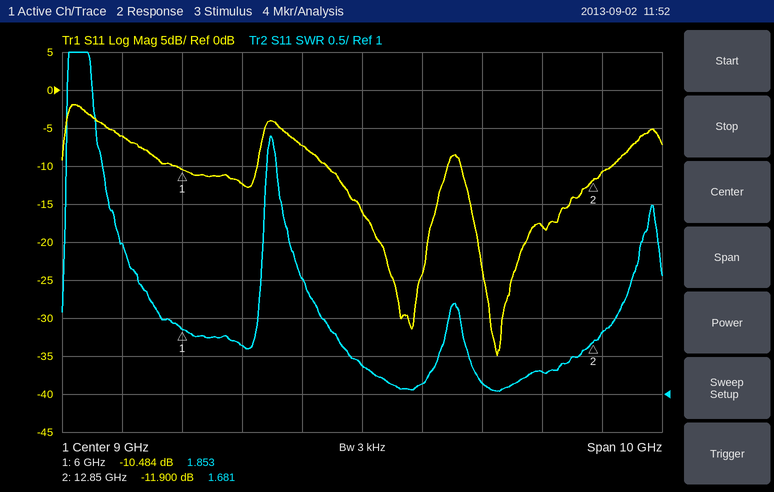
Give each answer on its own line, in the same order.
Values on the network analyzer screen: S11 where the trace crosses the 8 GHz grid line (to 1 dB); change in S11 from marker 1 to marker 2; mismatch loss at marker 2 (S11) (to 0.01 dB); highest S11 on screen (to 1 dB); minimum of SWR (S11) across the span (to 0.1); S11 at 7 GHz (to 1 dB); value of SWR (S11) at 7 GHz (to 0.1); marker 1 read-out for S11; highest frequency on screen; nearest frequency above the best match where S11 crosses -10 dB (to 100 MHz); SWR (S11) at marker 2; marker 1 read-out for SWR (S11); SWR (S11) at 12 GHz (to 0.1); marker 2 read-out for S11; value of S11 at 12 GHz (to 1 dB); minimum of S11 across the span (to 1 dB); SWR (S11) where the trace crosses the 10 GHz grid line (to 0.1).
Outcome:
-7 dB
-1.416 dB
0.29 dB
-2 dB
1.0
-12 dB
1.6
-10.484 dB
14 GHz
13.2 GHz
1.681
1.853
1.3
-11.900 dB
-18 dB
-35 dB
1.1
